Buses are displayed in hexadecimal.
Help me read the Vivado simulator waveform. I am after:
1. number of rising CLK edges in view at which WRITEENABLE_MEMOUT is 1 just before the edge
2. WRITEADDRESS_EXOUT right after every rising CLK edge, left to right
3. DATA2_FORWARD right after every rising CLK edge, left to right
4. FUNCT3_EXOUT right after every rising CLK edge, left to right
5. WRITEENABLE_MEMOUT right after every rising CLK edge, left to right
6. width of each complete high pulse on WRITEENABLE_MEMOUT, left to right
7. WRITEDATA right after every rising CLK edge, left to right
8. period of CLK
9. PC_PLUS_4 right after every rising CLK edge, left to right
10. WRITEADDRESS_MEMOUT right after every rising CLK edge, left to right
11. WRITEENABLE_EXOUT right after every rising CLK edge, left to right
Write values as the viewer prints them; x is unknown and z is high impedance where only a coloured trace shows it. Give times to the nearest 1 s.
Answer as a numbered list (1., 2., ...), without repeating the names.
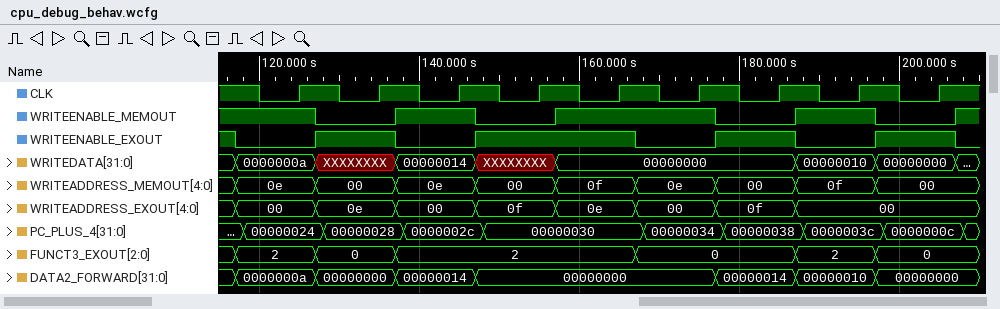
1. 5
2. 00, 0e, 00, 0f, 0e, 00, 0f, 00, 00
3. 0000000a, 00000000, 00000014, 00000000, 00000000, 00000000, 00000014, 00000010, 00000000
4. 2, 0, 2, 2, 2, 0, 0, 2, 0
5. 1 0 1 0 1 1 0 1 0
6. 10 s, 20 s, 10 s
7. 0000000a, XXXXXXXX, 00000014, XXXXXXXX, 00000000, 00000000, 00000000, 00000010, 00000000
8. 10 s
9. 00000024, 00000028, 0000002c, 00000030, 00000030, 00000034, 00000038, 0000003c, 0000000c
10. 0e, 00, 0e, 00, 0f, 0e, 00, 0f, 00
11. 0 1 0 1 1 0 1 0 1
